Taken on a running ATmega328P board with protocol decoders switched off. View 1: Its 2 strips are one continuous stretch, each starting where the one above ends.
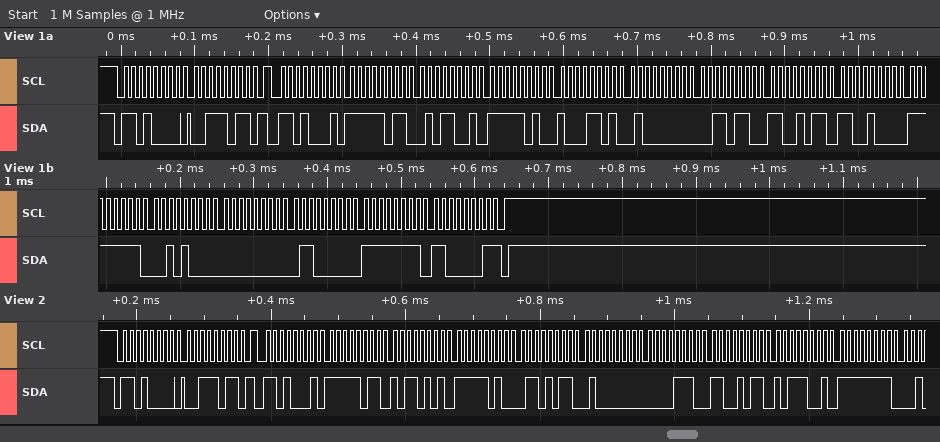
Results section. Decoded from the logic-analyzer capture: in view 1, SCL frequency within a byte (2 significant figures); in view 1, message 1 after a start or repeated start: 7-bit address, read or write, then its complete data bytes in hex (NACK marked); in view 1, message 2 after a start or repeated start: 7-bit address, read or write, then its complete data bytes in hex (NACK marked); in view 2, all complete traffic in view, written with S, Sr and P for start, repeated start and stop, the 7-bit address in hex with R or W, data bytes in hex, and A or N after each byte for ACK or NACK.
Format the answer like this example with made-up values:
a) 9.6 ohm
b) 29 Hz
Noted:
a) 100 kHz
b) 0x68 write: 3B
c) 0x68 read: FB 59 FA 8D 40 36 CB C8 FF 28 00 60 FF C1 NACK
d) S 68W A 3B A Sr 68R A FB A B5 A FA A 6B A 40 A 0E A CB A B9 A FF A
